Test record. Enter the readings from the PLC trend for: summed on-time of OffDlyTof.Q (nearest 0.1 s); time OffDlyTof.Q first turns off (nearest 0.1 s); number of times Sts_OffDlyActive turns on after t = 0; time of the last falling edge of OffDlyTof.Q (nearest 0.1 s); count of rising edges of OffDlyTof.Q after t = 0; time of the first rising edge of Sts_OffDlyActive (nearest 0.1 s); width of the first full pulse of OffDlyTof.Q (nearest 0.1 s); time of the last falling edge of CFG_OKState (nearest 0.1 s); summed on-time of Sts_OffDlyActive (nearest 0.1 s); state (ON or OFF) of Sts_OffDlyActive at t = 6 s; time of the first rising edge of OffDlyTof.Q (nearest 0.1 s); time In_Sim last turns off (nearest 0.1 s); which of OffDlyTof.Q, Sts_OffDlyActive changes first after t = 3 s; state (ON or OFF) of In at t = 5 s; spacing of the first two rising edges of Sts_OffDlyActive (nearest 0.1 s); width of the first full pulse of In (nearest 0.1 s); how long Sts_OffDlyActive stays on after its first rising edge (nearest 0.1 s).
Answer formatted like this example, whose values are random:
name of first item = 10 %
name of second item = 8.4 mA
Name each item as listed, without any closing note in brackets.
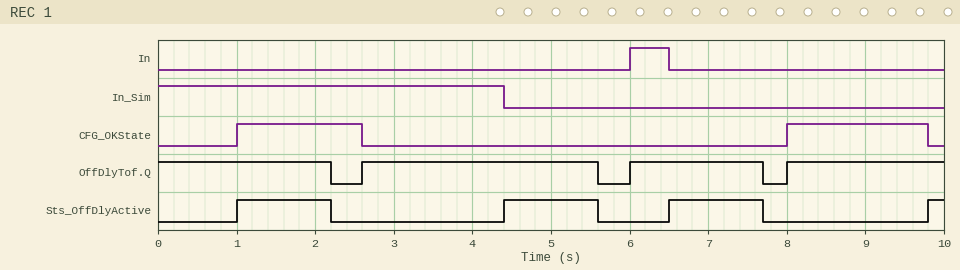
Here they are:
summed on-time of OffDlyTof.Q = 8.9 s
time OffDlyTof.Q first turns off = 2.2 s
number of times Sts_OffDlyActive turns on after t = 0 = 4
time of the last falling edge of OffDlyTof.Q = 7.7 s
count of rising edges of OffDlyTof.Q after t = 0 = 3
time of the first rising edge of Sts_OffDlyActive = 1.0 s
width of the first full pulse of OffDlyTof.Q = 3.0 s
time of the last falling edge of CFG_OKState = 9.8 s
summed on-time of Sts_OffDlyActive = 3.8 s
state (ON or OFF) of Sts_OffDlyActive at t = 6 s = OFF
time of the first rising edge of OffDlyTof.Q = 2.6 s
time In_Sim last turns off = 4.4 s
which of OffDlyTof.Q, Sts_OffDlyActive changes first after t = 3 s = Sts_OffDlyActive
state (ON or OFF) of In at t = 5 s = OFF
spacing of the first two rising edges of Sts_OffDlyActive = 3.4 s
width of the first full pulse of In = 0.5 s
how long Sts_OffDlyActive stays on after its first rising edge = 1.2 s
